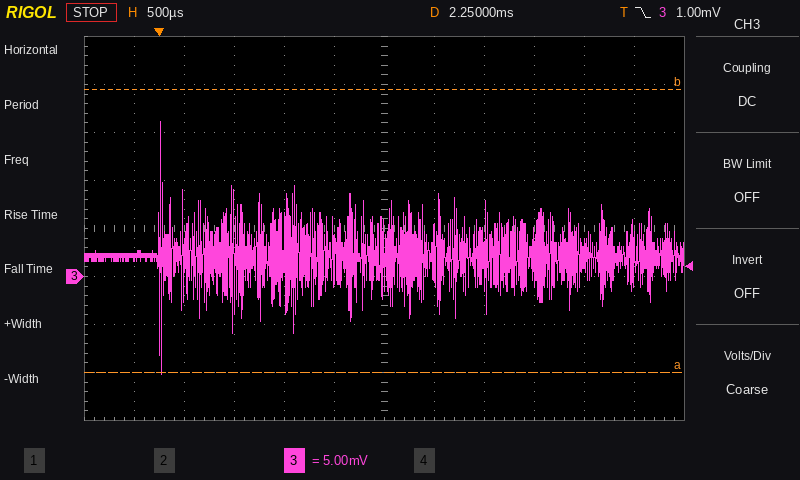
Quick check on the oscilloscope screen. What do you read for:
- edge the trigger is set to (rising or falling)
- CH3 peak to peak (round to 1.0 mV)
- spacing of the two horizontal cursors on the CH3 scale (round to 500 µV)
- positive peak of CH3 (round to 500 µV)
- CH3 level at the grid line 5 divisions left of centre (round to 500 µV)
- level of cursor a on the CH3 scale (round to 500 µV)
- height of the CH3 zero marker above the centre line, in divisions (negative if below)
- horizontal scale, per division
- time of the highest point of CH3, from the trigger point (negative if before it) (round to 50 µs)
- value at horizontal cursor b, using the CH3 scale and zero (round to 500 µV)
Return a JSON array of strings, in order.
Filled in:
["falling", "26.0 mV", "29.5 mV", "16.0 mV", "2.0 mV", "-10.0 mV", "-1.0 div", "500 µs", "0 µs", "19.5 mV"]
